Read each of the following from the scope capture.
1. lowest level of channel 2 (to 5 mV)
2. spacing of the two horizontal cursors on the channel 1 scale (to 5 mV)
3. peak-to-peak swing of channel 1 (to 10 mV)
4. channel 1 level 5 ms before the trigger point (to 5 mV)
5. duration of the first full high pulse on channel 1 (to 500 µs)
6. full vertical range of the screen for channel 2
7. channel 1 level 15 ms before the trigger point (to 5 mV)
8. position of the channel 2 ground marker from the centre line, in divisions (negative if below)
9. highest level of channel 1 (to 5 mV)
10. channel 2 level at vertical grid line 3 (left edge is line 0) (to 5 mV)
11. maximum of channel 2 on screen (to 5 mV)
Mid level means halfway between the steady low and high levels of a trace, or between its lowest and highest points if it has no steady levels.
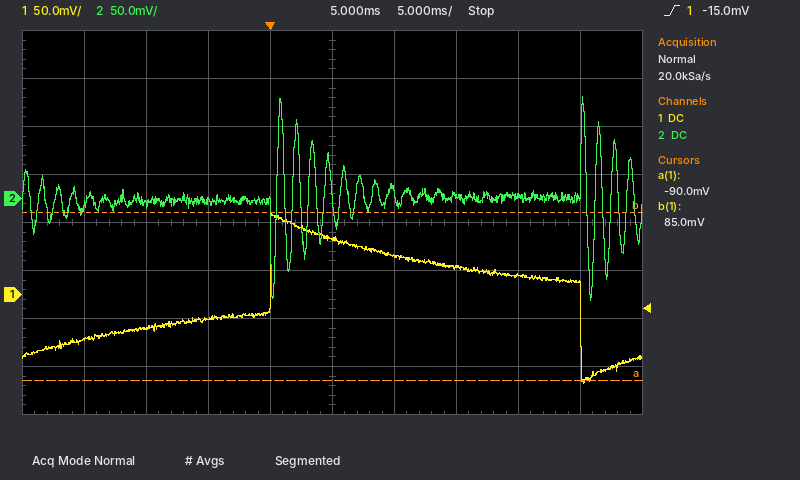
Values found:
-105 mV
175 mV
180 mV
-25 mV
25.0 ms
400 mV
-45 mV
+0.5 div
85 mV
-5 mV
105 mV
